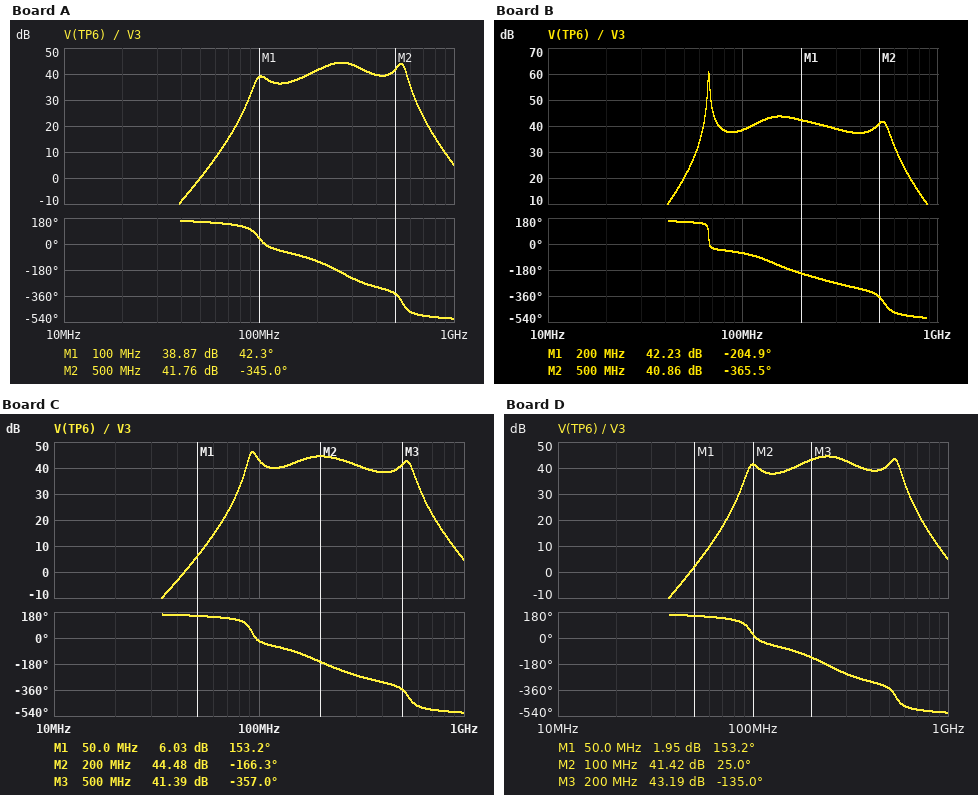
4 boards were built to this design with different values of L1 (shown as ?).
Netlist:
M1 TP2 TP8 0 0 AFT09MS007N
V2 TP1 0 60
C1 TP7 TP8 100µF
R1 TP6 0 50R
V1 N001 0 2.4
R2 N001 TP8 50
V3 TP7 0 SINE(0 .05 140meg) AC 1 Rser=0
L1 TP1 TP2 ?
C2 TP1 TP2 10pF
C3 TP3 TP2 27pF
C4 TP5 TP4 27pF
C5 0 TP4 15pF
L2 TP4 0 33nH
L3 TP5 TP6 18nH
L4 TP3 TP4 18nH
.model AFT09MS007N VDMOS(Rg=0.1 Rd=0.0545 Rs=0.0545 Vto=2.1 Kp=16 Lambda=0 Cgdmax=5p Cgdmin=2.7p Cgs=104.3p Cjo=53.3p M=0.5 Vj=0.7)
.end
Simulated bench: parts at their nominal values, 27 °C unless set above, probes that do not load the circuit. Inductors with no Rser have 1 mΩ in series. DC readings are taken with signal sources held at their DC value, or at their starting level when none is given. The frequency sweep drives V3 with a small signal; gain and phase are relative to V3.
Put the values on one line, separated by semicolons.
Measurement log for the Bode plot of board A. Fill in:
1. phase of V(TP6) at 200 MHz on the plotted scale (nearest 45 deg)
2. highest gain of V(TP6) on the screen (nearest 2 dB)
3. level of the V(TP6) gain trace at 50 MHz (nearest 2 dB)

-135 deg; 44 dB; 0 dB
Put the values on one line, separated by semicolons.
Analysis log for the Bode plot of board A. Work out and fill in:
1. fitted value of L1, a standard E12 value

18 nH
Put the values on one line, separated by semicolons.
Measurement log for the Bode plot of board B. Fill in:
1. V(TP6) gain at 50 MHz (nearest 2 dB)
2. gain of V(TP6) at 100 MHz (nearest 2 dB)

20 dB; 38 dB
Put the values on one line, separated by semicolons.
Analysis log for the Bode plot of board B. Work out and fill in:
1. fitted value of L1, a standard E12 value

100 nH
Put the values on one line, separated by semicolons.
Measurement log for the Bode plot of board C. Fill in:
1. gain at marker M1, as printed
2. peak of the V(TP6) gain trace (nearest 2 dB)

6.03 dB; 46 dB
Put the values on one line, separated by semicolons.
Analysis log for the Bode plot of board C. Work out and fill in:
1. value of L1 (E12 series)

33 nH
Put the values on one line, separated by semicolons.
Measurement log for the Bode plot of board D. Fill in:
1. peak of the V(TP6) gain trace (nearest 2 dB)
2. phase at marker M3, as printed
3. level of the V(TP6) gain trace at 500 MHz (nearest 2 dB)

44 dB; -135.0 deg; 42 dB
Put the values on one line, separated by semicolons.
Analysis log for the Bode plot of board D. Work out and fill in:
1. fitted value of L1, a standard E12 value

22 nH
